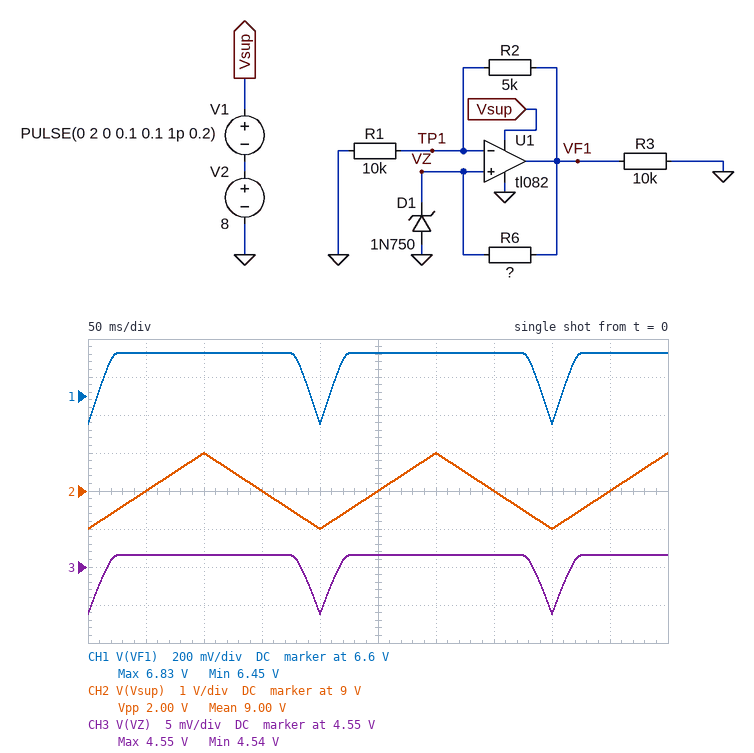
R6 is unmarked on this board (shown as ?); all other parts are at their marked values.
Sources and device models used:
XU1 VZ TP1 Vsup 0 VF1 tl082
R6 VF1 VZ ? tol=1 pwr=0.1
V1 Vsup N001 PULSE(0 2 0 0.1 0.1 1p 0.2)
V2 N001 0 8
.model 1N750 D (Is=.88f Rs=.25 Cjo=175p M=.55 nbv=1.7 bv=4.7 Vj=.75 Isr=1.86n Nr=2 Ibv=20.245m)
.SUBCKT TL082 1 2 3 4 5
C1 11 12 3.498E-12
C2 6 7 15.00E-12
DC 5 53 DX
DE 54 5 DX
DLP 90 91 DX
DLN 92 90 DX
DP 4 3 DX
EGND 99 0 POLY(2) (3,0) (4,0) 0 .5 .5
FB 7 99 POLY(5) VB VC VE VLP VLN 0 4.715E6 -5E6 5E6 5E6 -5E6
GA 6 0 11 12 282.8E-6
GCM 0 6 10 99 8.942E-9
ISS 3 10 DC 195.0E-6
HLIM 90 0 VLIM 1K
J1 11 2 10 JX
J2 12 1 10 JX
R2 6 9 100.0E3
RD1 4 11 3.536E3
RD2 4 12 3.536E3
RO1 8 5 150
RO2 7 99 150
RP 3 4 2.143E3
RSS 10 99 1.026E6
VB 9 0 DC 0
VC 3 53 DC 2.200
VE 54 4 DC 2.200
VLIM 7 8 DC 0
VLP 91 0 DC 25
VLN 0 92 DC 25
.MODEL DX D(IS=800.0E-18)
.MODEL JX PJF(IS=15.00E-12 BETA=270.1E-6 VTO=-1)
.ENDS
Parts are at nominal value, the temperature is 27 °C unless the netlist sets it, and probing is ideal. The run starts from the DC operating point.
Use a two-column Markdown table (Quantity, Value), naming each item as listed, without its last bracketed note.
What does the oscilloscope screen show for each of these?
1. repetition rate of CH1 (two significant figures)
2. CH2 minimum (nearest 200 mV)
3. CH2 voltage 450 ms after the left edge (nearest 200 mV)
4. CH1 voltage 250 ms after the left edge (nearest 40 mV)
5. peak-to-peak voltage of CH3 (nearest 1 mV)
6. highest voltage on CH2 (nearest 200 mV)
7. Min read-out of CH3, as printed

| Quantity | Value |
|---|---|
| repetition rate of CH1 | 5.0 Hz |
| CH2 minimum | 8.0 V |
| CH2 voltage 450 ms after the left edge | 9.0 V |
| CH1 voltage 250 ms after the left edge | 6.84 V |
| peak-to-peak voltage of CH3 | 8 mV |
| highest voltage on CH2 | 10.0 V |
| Min read-out of CH3, as printed | 4.54 V |
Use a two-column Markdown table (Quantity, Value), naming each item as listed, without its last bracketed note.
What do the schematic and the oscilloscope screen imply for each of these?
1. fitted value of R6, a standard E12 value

| Quantity | Value |
|---|---|
| fitted value of R6, a standard E12 value | 3.3 kΩ |
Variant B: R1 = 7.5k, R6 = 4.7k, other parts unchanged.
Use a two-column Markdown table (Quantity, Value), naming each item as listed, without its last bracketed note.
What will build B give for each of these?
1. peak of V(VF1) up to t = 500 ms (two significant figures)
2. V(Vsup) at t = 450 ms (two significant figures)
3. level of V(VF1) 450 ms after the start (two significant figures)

| Quantity | Value |
|---|---|
| peak of V(VF1) up to t = 500 ms | 7.6 V |
| V(Vsup) at t = 450 ms | 9.0 V |
| level of V(VF1) 450 ms after the start | 7.4 V |
